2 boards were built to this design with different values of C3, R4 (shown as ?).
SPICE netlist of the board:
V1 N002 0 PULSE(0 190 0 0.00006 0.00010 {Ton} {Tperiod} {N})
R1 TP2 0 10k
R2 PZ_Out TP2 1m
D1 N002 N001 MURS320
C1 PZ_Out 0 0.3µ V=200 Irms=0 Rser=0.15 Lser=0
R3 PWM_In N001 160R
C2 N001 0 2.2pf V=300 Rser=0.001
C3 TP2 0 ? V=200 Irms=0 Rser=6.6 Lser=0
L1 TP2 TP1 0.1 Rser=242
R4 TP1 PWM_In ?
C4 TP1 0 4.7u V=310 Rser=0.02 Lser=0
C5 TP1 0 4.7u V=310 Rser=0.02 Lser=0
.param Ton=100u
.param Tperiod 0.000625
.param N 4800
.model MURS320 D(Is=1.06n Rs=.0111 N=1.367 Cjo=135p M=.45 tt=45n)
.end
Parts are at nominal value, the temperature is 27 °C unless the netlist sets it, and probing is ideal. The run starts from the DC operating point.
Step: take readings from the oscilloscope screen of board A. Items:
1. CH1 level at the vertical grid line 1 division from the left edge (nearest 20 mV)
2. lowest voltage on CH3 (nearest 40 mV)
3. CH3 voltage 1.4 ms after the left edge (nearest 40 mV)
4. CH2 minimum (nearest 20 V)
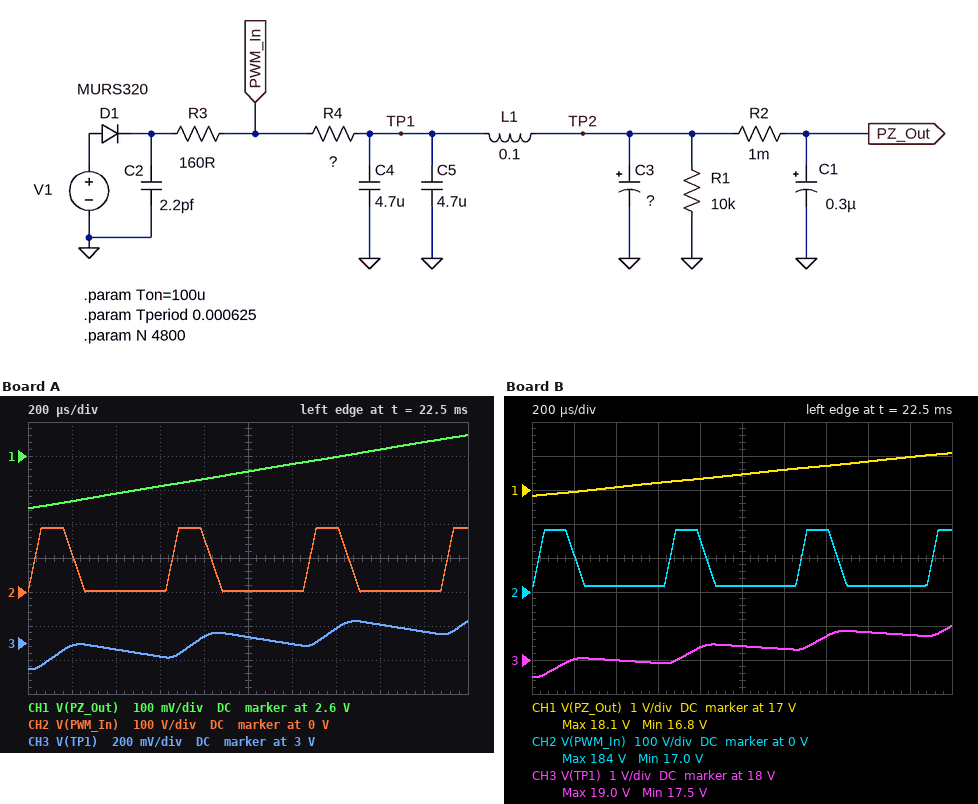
2.46 V
2.84 V
3.08 V
0 V
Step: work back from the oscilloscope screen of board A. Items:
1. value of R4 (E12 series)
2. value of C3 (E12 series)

18 kΩ
15 µF
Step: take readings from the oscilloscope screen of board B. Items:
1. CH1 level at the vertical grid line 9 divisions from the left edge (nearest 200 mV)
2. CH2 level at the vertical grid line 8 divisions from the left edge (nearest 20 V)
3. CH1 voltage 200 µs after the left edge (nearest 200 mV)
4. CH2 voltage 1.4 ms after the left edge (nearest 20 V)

18.0 V
20 V
17.0 V
180 V
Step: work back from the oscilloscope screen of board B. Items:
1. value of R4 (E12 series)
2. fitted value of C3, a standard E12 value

4.7 kΩ
2.7 µF
